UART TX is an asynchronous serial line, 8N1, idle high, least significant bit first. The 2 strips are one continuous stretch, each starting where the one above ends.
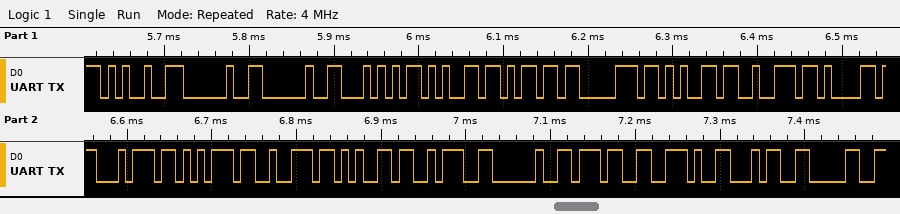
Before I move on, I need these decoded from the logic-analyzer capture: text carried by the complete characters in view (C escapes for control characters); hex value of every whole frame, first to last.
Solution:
"%  Temperature: 7.40"
25 20 20 54 65 6D 70 65 72 61 74 75 72 65 3A 20 37 2E 34 30
